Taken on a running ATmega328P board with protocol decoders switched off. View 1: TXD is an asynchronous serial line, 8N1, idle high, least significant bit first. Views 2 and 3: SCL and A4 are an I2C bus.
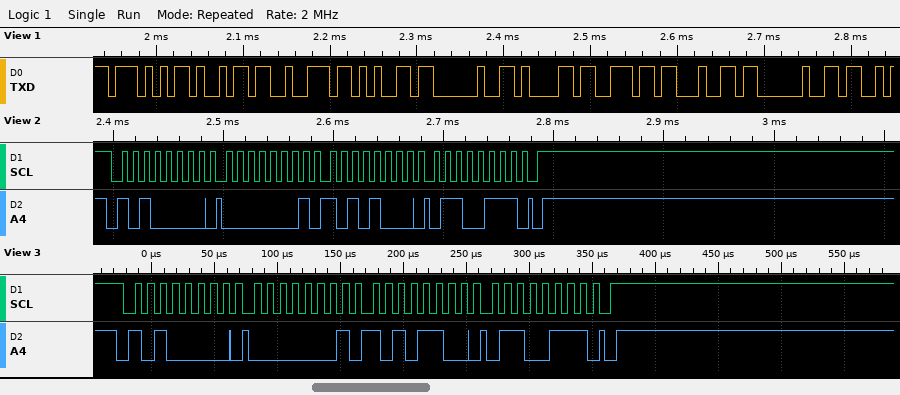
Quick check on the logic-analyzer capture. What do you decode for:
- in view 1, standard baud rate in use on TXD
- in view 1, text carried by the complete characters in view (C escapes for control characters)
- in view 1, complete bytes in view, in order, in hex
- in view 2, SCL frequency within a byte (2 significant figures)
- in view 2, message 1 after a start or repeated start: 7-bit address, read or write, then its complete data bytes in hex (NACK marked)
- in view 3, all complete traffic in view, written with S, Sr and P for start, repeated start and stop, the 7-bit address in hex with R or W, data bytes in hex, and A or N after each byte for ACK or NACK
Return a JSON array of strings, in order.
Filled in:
["115200 baud", "\"Wire and \"", "57 69 72 65 20 61 6E 64 20", "100 kHz", "0x50 write: 01 A8 67", "S 50W A 01 A AC A 67 A P"]
